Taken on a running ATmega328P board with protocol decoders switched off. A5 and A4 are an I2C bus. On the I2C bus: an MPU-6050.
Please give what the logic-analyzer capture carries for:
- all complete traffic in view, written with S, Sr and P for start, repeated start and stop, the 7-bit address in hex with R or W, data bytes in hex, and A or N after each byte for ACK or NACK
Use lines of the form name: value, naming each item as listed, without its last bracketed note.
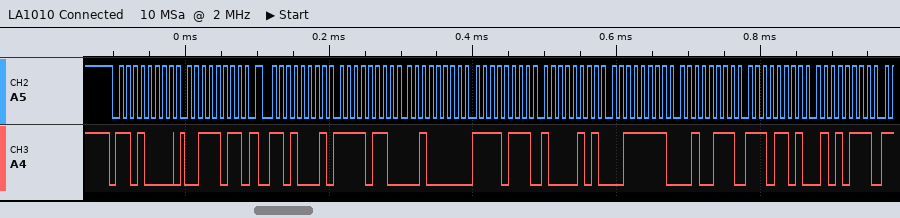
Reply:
all complete traffic in view, written with S, Sr and P for start, repeated start and stop, the 7-bit address in hex with R or W, data bytes in hex, and A or N after each byte for ACK or NACK: S 68W A 3B A Sr 68R A F6 A 20 A F7 A 85 A 3F A 27 A ED A 57 A
